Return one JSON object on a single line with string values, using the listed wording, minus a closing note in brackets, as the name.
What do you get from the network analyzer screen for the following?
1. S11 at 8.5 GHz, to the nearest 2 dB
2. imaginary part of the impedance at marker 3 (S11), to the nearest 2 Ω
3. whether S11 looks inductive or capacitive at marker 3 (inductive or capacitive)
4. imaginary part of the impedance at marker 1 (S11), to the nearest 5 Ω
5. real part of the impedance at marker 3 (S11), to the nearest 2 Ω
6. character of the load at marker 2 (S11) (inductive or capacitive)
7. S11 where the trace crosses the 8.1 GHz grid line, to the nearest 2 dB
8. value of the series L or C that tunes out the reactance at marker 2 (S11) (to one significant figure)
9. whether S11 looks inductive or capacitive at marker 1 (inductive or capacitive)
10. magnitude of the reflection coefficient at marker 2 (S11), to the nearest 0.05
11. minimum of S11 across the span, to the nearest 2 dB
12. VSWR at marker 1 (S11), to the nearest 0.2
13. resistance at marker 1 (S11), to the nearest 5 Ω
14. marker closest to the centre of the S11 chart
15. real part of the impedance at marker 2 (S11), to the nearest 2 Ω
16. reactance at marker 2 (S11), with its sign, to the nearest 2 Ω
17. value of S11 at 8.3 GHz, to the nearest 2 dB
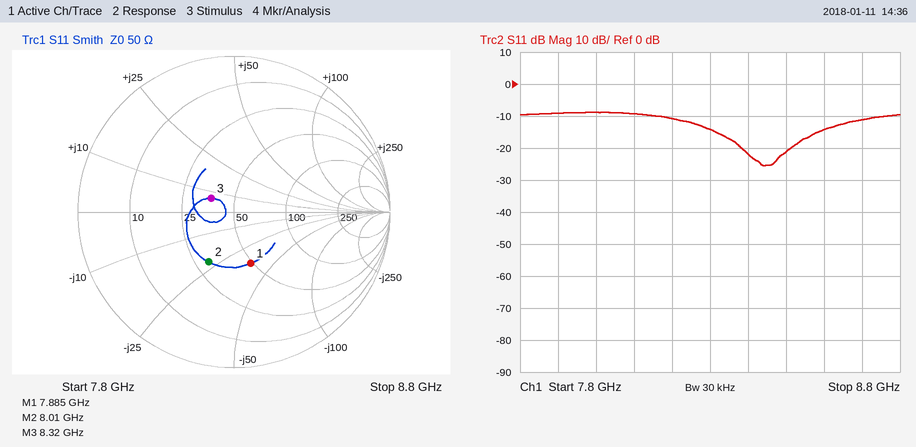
{"S11 at 8.5 GHz, to the nearest 2 dB": "-22 dB", "imaginary part of the impedance at marker 3 (S11), to the nearest 2 Ω": "+6 Ω", "whether S11 looks inductive or capacitive at marker 3": "inductive", "imaginary part of the impedance at marker 1 (S11), to the nearest 5 Ω": "-35 Ω", "real part of the impedance at marker 3 (S11), to the nearest 2 Ω": "36 Ω", "character of the load at marker 2 (S11)": "capacitive", "S11 where the trace crosses the 8.1 GHz grid line, to the nearest 2 dB": "-10 dB", "value of the series L or C that tunes out the reactance at marker 2 (S11)": "400 pH", "whether S11 looks inductive or capacitive at marker 1": "capacitive", "magnitude of the reflection coefficient at marker 2 (S11), to the nearest 0.05": "0.35", "minimum of S11 across the span, to the nearest 2 dB": "-26 dB", "VSWR at marker 1 (S11), to the nearest 0.2": "2.0", "resistance at marker 1 (S11), to the nearest 5 Ω": "50 Ω", "marker closest to the centre of the S11 chart": "marker 3", "real part of the impedance at marker 2 (S11), to the nearest 2 Ω": "30 Ω", "reactance at marker 2 (S11), with its sign, to the nearest 2 Ω": "-22 Ω", "value of S11 at 8.3 GHz, to the nearest 2 dB": "-14 dB"}
